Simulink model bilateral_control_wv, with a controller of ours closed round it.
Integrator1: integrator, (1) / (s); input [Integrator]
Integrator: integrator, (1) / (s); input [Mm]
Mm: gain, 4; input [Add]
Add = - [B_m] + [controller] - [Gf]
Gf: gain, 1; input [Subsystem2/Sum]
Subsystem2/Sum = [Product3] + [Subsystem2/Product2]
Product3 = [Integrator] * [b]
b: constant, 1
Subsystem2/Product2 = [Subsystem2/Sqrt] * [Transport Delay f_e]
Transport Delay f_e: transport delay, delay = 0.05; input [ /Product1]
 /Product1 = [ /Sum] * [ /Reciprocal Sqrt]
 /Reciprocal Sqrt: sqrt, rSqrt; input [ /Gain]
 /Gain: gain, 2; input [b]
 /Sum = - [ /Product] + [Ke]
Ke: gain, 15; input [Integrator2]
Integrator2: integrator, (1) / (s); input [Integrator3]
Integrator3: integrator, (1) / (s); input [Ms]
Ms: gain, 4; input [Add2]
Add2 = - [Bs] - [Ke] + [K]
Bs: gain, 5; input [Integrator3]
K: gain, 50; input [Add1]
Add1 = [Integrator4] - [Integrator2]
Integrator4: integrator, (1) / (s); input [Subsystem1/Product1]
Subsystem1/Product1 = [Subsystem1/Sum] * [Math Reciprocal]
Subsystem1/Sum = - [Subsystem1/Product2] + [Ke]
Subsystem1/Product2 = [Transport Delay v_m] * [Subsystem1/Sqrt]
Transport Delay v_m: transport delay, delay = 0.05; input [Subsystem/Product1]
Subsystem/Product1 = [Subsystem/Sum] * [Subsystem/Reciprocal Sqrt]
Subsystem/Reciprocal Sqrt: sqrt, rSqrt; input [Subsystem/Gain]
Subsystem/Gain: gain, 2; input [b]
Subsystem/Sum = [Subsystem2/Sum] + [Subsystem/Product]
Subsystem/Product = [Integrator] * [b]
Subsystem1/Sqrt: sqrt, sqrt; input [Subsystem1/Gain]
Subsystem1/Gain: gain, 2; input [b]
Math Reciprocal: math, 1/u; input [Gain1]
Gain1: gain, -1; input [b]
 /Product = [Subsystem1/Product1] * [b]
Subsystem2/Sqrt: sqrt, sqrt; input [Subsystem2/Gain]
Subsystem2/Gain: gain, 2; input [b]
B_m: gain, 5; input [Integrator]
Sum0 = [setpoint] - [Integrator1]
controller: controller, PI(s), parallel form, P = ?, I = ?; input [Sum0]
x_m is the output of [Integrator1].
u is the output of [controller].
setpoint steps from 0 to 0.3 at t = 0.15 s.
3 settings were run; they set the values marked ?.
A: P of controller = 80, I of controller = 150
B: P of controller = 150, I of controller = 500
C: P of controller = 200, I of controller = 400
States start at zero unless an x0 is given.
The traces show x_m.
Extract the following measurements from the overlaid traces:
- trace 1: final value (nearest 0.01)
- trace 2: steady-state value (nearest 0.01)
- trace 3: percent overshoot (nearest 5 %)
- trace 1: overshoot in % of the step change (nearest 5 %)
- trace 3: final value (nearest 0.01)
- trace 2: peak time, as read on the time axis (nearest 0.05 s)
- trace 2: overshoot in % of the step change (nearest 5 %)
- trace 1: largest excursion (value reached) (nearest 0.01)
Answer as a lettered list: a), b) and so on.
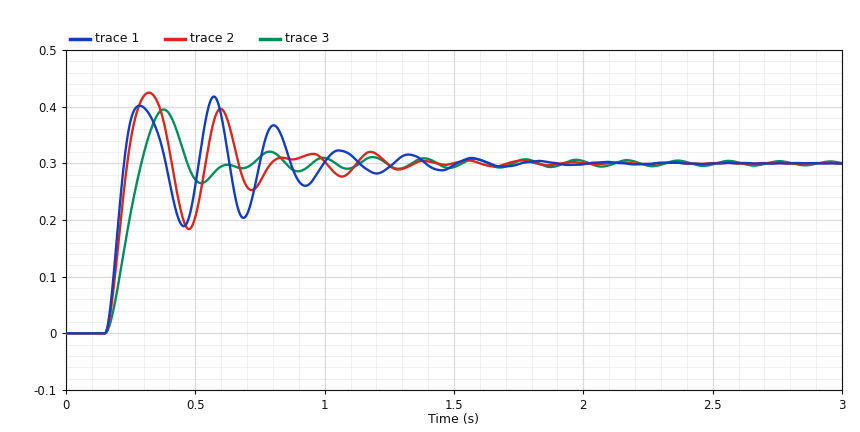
a) 0.30
b) 0.30
c) 30 %
d) 40 %
e) 0.30
f) 0.30 s
g) 40 %
h) 0.42
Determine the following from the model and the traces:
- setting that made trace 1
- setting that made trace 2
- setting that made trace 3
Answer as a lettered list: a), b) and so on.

a) C
b) B
c) A
